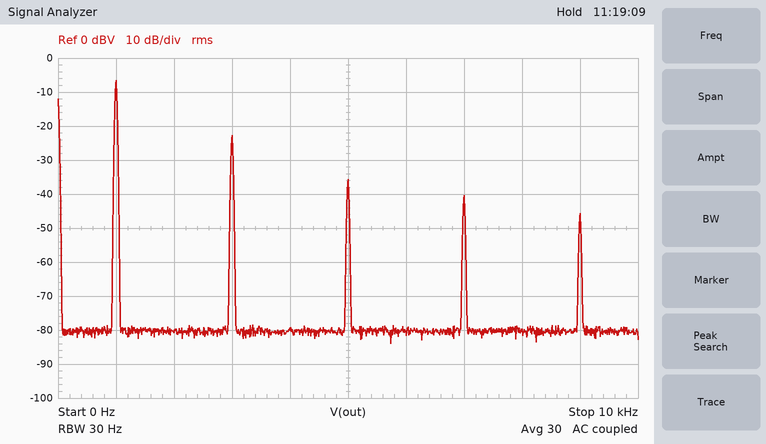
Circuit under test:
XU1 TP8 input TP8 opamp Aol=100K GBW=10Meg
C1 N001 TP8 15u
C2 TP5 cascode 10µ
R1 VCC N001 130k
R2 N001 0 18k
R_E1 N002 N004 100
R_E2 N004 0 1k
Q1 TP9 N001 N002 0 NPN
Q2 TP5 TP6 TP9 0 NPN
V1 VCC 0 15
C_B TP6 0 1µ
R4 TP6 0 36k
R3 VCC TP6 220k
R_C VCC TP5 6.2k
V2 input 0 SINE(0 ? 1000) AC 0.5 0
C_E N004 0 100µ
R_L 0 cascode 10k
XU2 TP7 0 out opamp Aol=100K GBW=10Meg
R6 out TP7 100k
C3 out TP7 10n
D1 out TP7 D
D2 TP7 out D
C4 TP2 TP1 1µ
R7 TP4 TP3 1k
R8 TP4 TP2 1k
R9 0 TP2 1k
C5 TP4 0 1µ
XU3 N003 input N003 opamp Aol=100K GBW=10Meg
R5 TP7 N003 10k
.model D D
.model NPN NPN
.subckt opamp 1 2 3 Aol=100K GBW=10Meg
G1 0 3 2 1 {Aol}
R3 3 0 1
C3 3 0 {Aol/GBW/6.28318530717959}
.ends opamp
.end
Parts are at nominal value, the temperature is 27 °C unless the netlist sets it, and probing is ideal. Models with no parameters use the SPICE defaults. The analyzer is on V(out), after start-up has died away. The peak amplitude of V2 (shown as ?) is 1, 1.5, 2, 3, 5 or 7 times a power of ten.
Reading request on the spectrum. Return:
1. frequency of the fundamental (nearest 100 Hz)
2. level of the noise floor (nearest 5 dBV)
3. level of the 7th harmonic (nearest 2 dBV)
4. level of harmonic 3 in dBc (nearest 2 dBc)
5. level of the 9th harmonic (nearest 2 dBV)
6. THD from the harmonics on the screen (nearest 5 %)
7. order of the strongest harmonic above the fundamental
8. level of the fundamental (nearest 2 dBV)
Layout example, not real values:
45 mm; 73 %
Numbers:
1.0 kHz; -80 dBV; -40 dBV; -16 dBc; -46 dBV; 15 %; 3; -6 dBV
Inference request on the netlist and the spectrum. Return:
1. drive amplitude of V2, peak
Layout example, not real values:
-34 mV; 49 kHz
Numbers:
700 mV
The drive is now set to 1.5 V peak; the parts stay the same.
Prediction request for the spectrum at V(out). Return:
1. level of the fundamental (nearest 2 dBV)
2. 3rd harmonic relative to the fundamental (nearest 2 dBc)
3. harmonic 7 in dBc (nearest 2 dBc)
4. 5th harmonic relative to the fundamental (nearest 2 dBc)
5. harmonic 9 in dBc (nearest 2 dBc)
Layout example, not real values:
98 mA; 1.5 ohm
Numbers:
-6 dBV; -12 dBc; -30 dBc; -22 dBc; -34 dBc
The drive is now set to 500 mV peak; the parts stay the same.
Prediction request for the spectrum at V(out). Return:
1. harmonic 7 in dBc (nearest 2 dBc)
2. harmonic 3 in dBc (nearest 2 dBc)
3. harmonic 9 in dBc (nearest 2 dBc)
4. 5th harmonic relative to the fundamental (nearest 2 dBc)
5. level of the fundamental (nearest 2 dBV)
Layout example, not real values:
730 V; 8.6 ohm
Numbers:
-38 dBc; -20 dBc; -42 dBc; -32 dBc; -8 dBV
